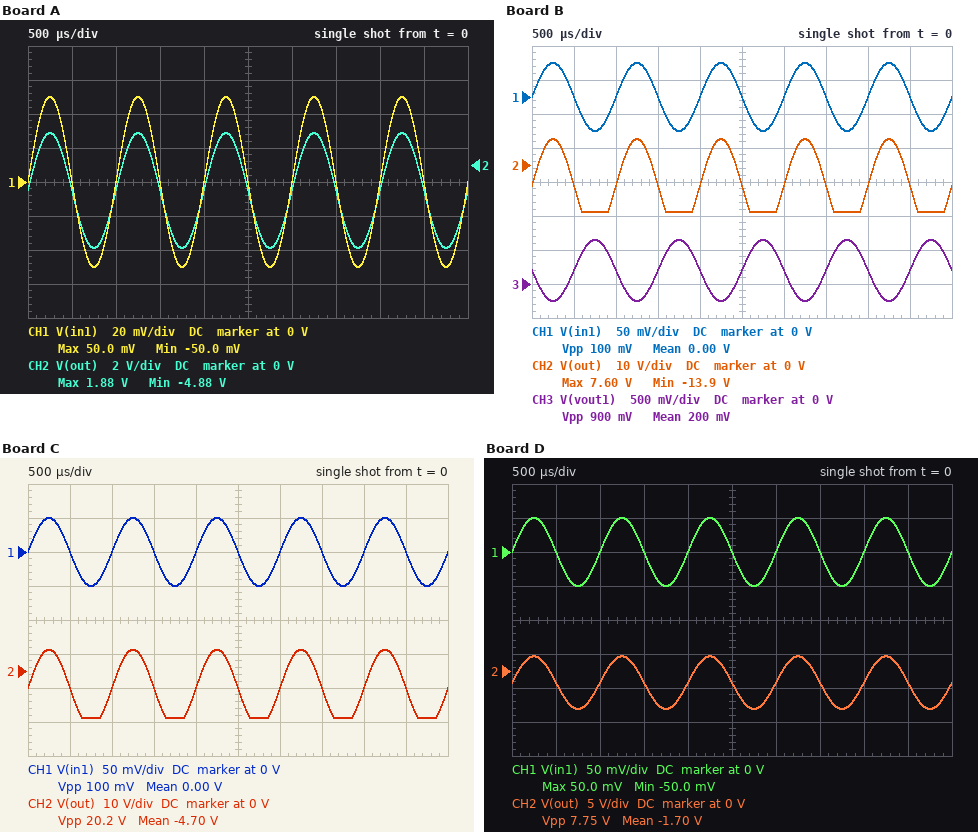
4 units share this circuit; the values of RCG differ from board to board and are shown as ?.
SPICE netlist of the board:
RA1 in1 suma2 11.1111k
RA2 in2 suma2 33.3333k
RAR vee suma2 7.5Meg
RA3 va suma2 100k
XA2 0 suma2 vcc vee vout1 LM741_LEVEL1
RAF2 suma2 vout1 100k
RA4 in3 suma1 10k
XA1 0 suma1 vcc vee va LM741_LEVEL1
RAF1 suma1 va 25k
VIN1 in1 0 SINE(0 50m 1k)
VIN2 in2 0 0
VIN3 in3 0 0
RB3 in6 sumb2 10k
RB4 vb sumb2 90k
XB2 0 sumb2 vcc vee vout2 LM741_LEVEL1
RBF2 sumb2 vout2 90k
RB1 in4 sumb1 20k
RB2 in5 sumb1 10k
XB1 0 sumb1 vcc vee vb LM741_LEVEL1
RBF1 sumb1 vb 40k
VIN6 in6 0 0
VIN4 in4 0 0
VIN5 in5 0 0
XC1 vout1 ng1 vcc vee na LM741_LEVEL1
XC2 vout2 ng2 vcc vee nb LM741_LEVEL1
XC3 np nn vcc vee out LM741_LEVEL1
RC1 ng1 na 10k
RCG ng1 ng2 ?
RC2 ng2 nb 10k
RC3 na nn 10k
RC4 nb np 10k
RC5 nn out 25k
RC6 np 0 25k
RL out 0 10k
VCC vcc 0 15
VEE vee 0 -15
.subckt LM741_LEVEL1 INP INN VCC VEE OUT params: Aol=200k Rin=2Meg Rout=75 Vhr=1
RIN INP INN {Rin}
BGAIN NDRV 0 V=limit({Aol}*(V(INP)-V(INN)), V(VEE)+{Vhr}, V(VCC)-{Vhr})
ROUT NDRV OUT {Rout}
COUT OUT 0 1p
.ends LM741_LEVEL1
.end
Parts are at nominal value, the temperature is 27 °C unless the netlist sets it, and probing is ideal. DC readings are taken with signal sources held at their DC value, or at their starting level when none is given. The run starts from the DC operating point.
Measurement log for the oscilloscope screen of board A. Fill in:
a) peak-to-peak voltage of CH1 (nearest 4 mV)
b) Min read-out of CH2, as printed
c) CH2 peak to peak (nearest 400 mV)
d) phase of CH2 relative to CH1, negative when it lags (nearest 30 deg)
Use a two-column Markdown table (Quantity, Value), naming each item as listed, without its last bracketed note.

| Quantity | Value |
|---|---|
| peak-to-peak voltage of CH1 | 100 mV |
| Min read-out of CH2, as printed | -4.88 V |
| CH2 peak to peak | 6.8 V |
| phase of CH2 relative to CH1, negative when it lags | 0 deg |
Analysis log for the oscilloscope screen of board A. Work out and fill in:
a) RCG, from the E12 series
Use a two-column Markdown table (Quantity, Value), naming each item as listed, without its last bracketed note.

| Quantity | Value |
|---|---|
| RCG, from the E12 series | 10 kΩ |
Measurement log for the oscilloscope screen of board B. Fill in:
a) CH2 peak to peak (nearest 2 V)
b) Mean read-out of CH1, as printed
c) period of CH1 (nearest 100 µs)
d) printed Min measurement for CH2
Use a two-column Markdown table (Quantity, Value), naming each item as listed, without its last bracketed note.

| Quantity | Value |
|---|---|
| CH2 peak to peak | 22 V |
| Mean read-out of CH1, as printed | 0.00 V |
| period of CH1 | 1.0 ms |
| printed Min measurement for CH2 | -13.9 V |
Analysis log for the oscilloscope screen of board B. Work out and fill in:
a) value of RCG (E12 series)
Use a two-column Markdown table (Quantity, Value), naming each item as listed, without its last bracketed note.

| Quantity | Value |
|---|---|
| value of RCG | 1.8 kΩ |
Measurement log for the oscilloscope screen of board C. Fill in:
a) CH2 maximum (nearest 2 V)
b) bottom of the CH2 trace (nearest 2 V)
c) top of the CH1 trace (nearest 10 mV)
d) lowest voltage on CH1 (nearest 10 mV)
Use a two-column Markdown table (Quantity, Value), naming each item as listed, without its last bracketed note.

| Quantity | Value |
|---|---|
| CH2 maximum | 6 V |
| bottom of the CH2 trace | -14 V |
| top of the CH1 trace | 50 mV |
| lowest voltage on CH1 | -50 mV |
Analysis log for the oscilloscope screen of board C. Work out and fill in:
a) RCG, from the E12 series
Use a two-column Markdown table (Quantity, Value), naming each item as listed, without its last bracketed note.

| Quantity | Value |
|---|---|
| RCG, from the E12 series | 2.2 kΩ |
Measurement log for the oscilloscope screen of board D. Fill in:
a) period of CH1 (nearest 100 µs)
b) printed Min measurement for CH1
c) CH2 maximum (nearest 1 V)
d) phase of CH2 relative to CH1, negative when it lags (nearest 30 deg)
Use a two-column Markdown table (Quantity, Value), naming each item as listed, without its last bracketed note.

| Quantity | Value |
|---|---|
| period of CH1 | 1.0 ms |
| printed Min measurement for CH1 | -50.0 mV |
| CH2 maximum | 2 V |
| phase of CH2 relative to CH1, negative when it lags | 0 deg |
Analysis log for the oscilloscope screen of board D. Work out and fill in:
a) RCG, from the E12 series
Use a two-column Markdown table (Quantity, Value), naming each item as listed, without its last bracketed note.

| Quantity | Value |
|---|---|
| RCG, from the E12 series | 8.2 kΩ |
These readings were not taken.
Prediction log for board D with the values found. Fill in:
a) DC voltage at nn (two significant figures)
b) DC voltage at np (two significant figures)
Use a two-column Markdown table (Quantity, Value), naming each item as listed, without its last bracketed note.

| Quantity | Value |
|---|---|
| DC voltage at nn | -170 mV |
| DC voltage at np | -170 mV |
